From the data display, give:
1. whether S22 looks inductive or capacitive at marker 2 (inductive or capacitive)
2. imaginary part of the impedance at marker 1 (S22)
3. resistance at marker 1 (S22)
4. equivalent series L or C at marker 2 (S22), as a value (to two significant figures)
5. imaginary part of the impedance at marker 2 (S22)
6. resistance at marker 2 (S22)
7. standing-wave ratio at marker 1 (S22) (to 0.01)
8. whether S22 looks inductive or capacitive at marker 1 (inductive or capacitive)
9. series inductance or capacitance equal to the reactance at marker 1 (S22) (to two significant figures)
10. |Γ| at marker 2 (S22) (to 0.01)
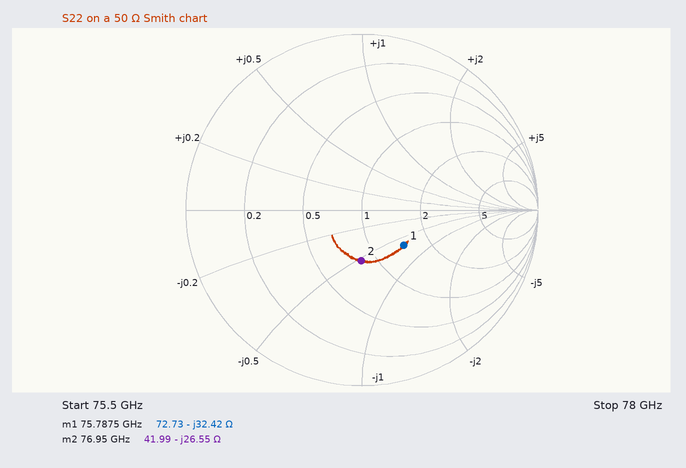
capacitive
-32.42 Ω
72.73 Ω
78 fF
-26.55 Ω
41.99 Ω
1.91
capacitive
65 fF
0.29
